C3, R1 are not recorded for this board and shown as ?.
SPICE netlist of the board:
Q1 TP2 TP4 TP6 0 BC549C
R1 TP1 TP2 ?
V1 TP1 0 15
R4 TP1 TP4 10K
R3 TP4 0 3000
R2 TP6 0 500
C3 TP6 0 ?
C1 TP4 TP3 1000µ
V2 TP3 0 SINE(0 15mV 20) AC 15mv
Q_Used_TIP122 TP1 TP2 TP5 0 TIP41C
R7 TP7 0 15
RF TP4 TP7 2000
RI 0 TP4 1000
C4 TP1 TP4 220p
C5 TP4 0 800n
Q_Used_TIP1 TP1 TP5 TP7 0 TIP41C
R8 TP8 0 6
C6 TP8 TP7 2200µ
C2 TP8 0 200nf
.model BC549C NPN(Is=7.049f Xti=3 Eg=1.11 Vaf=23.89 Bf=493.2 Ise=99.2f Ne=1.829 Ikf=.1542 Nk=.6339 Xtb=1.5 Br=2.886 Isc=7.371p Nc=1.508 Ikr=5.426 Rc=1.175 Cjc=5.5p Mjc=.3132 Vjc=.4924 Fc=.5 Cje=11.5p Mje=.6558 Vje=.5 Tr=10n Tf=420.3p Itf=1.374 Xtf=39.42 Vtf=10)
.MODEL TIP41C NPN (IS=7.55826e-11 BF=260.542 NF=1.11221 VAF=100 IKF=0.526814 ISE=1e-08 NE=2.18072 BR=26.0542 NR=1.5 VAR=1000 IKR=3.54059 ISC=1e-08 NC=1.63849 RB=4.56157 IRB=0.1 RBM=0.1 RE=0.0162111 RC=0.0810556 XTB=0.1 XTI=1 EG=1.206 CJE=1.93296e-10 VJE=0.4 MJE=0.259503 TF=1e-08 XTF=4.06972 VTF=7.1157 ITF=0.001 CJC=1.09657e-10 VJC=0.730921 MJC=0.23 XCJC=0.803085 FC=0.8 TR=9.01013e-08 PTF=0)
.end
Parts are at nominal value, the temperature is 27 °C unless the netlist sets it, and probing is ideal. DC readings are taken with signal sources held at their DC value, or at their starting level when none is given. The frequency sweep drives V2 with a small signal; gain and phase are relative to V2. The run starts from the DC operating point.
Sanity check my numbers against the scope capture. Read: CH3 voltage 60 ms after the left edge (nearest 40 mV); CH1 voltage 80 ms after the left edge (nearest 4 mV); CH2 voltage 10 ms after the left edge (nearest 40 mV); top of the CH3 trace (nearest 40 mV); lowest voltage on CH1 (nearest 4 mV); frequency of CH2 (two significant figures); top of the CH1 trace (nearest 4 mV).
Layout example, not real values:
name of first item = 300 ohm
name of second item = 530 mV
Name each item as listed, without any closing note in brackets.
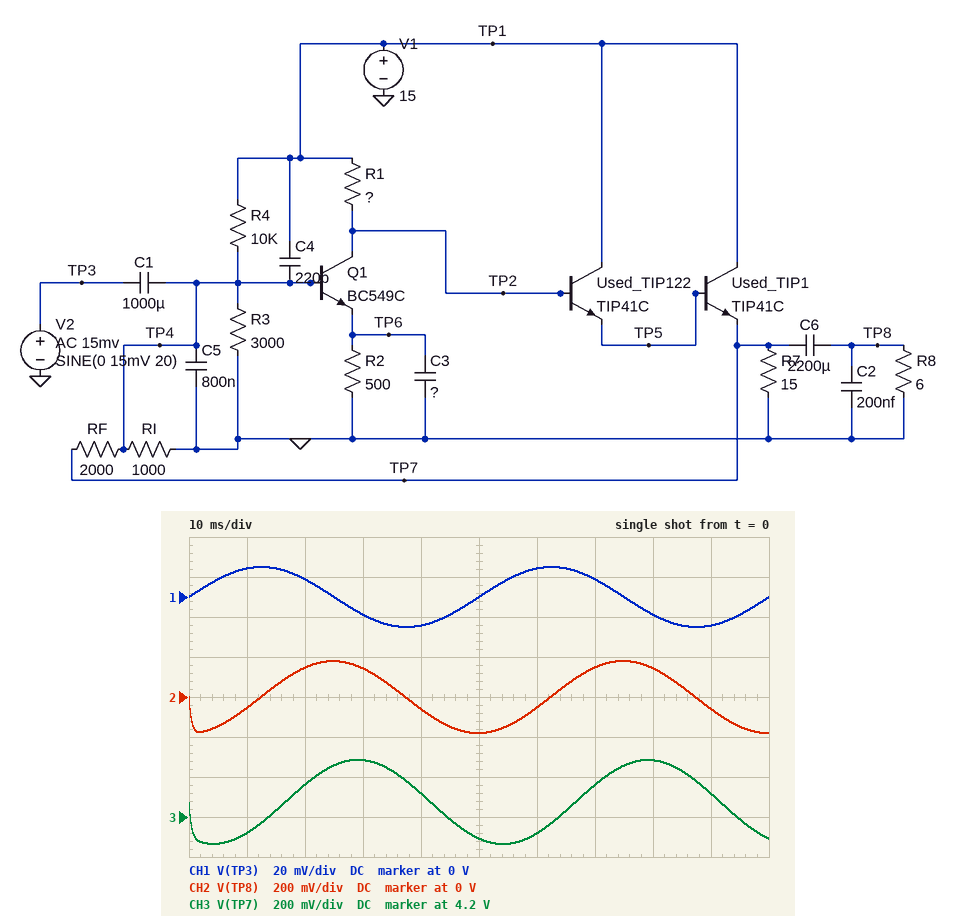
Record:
CH3 voltage 60 ms after the left edge = 4.12 V
CH1 voltage 80 ms after the left edge = -8 mV
CH2 voltage 10 ms after the left edge = -40 mV
top of the CH3 trace = 4.48 V
lowest voltage on CH1 = -16 mV
frequency of CH2 = 20 Hz
top of the CH1 trace = 16 mV
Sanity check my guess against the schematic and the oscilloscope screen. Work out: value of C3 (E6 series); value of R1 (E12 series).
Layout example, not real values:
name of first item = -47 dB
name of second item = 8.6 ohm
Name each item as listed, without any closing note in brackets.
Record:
value of C3 = 33 µF
value of R1 = 3.9 kΩ
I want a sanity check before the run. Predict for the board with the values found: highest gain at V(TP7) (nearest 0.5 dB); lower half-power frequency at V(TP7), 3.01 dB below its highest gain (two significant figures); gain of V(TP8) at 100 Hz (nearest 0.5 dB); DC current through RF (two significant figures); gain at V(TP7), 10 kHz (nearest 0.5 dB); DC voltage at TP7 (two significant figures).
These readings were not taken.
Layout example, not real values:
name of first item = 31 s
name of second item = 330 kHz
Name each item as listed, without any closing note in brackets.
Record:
highest gain at V(TP7) = 53.5 dB
lower half-power frequency at V(TP7), 3.01 dB below its highest gain = 130 kHz
gain of V(TP8) at 100 Hz = 35.5 dB
DC current through RF = 1.2 mA
gain at V(TP7), 10 kHz = 47.0 dB
DC voltage at TP7 = 4.3 V
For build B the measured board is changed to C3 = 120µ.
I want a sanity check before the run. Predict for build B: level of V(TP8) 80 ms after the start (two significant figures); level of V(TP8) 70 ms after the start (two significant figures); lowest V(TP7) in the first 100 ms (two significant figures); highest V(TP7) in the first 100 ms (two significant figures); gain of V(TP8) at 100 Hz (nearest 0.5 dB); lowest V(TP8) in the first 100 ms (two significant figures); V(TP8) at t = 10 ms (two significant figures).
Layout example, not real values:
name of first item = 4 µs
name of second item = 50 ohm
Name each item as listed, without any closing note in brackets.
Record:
level of V(TP8) 80 ms after the start = 340 mV
level of V(TP8) 70 ms after the start = 470 mV
lowest V(TP7) in the first 100 ms = 3.7 V
highest V(TP7) in the first 100 ms = 4.9 V
gain of V(TP8) at 100 Hz = 43.5 dB
lowest V(TP8) in the first 100 ms = -520 mV
V(TP8) at t = 10 ms = -110 mV
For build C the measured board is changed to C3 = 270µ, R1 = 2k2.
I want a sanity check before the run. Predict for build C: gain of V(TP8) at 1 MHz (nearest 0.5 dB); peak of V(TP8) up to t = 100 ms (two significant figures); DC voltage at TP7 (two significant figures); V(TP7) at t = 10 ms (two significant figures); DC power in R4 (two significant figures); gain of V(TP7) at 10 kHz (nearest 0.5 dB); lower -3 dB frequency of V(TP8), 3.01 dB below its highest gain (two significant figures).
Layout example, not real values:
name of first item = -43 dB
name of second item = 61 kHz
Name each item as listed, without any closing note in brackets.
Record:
gain of V(TP8) at 1 MHz = 9.5 dB
peak of V(TP8) up to t = 100 ms = 640 mV
DC voltage at TP7 = 6.2 V
V(TP7) at t = 10 ms = 5.8 V
DC power in R4 = 16 mW
gain of V(TP7) at 10 kHz = 46.0 dB
lower -3 dB frequency of V(TP8), 3.01 dB below its highest gain = 180 kHz
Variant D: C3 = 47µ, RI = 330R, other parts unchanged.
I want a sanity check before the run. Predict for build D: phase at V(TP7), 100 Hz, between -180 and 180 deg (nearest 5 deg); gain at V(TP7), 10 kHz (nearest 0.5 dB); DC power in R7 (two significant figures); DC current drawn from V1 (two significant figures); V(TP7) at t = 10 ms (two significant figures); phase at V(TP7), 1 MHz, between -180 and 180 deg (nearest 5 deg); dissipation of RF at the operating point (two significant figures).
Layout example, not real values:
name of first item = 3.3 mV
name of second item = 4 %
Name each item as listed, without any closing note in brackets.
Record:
phase at V(TP7), 100 Hz, between -180 and 180 deg = -125 deg
gain at V(TP7), 10 kHz = 43.5 dB
DC power in R7 = 4.1 W
DC current drawn from V1 = 530 mA
V(TP7) at t = 10 ms = 7.7 V
phase at V(TP7), 1 MHz, between -180 and 180 deg = -45 deg
dissipation of RF at the operating point = 21 mW
